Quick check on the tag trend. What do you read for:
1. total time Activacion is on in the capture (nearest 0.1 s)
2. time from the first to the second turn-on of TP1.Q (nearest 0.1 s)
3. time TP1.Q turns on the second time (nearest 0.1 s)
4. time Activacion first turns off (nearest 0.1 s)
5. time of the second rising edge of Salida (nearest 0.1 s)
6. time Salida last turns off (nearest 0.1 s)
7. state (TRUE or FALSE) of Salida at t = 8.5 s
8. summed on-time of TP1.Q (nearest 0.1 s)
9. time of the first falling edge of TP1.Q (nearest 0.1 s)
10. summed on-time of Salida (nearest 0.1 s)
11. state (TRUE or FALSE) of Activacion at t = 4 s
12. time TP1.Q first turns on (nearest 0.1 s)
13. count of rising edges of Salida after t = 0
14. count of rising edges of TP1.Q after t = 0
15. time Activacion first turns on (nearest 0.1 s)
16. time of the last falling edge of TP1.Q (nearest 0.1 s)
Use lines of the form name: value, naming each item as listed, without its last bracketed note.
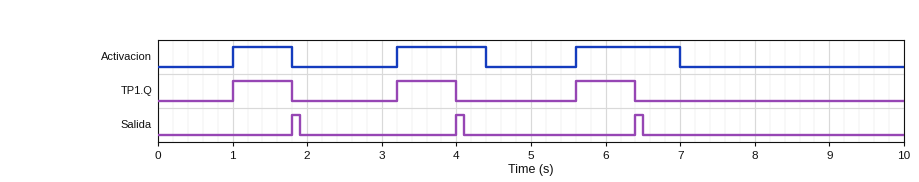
total time Activacion is on in the capture: 3.4 s
time from the first to the second turn-on of TP1.Q: 2.2 s
time TP1.Q turns on the second time: 3.2 s
time Activacion first turns off: 1.8 s
time of the second rising edge of Salida: 4.0 s
time Salida last turns off: 6.5 s
state (TRUE or FALSE) of Salida at t = 8.5 s: FALSE
summed on-time of TP1.Q: 2.4 s
time of the first falling edge of TP1.Q: 1.8 s
summed on-time of Salida: 0.3 s
state (TRUE or FALSE) of Activacion at t = 4 s: TRUE
time TP1.Q first turns on: 1.0 s
count of rising edges of Salida after t = 0: 3
count of rising edges of TP1.Q after t = 0: 3
time Activacion first turns on: 1.0 s
time of the last falling edge of TP1.Q: 6.4 s
